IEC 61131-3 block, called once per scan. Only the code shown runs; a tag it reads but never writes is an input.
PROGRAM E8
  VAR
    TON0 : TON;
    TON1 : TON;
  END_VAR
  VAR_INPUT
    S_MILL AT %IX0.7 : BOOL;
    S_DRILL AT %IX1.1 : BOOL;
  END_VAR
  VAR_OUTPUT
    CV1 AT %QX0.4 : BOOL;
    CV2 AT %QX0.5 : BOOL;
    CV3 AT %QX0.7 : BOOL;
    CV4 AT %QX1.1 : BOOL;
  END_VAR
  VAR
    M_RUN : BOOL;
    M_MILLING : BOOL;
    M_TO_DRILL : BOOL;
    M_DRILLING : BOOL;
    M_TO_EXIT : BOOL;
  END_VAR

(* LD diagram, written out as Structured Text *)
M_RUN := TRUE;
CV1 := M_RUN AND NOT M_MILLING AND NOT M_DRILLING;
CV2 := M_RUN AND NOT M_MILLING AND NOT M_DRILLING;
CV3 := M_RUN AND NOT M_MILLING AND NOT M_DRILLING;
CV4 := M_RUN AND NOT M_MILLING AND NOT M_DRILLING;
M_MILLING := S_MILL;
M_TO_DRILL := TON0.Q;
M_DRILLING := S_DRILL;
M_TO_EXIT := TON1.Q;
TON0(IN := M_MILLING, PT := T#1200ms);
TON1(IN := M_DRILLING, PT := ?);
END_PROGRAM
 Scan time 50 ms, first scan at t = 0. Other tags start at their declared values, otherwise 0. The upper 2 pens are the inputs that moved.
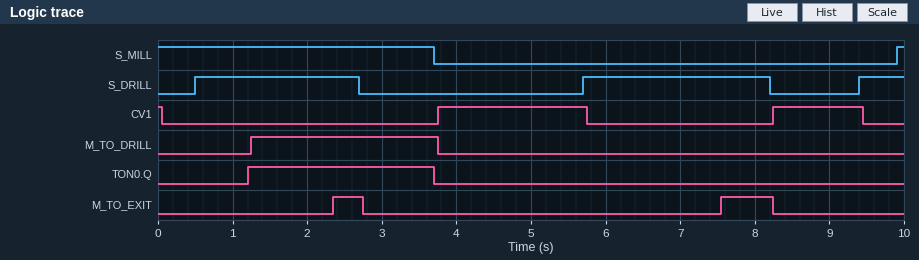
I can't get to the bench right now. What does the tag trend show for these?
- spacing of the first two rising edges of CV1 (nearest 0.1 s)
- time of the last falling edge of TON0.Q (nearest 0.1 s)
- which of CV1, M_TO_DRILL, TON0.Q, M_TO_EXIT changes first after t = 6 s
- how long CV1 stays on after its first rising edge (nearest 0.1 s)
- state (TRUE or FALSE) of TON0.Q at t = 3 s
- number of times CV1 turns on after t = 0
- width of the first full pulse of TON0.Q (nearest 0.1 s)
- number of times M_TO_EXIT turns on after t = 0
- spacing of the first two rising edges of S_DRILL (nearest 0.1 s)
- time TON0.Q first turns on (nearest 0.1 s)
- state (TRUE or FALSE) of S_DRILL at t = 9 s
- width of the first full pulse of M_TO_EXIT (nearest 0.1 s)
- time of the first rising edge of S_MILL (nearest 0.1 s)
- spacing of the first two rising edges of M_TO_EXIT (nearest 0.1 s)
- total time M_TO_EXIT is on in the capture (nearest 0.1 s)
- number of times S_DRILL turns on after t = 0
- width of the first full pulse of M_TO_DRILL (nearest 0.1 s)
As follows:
4.5 s
3.7 s
M_TO_EXIT
2.0 s
TRUE
2
2.5 s
2
5.2 s
1.2 s
FALSE
0.4 s
9.9 s
5.2 s
1.1 s
3
2.5 s
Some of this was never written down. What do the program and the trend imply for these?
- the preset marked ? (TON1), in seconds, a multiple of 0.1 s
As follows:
1.8 s
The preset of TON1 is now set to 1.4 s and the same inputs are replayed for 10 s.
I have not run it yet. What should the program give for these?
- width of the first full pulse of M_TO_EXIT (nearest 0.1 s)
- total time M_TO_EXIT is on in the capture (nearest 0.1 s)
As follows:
0.8 s
1.9 s
